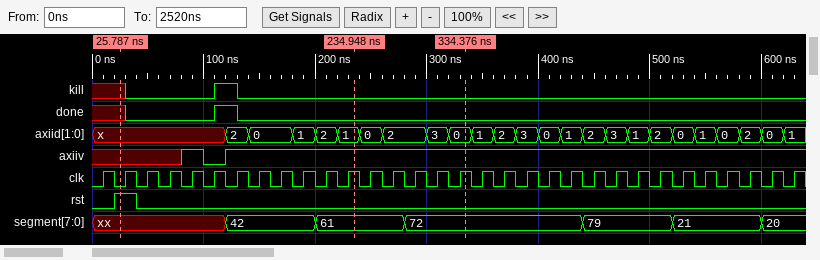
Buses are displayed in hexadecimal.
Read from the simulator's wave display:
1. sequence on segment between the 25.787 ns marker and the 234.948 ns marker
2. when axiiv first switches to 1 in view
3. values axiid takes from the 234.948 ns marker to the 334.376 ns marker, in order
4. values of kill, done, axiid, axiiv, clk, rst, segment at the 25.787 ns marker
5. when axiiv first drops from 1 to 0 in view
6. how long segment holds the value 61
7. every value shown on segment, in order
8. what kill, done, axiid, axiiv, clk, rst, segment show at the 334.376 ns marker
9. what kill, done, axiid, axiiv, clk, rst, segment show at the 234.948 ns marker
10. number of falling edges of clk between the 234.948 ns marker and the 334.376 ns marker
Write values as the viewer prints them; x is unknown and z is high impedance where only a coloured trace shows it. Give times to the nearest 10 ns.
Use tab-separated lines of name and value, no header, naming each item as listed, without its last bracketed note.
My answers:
sequence on segment between the 25.787 ns marker and the 234.948 ns marker	xx, 42, 61
when axiiv first switches to 1 in view	80 ns
values axiid takes from the 234.948 ns marker to the 334.376 ns marker, in order	1, 0, 2, 3, 0
values of kill, done, axiid, axiiv, clk, rst, segment at the 25.787 ns marker	kill=x, done=x, axiid=x, axiiv=x, clk=0, rst=1, segment=xx
when axiiv first drops from 1 to 0 in view	100 ns
how long segment holds the value 61	80 ns
every value shown on segment, in order	xx, 42, 61, 72, 79, 21, 20
what kill, done, axiid, axiiv, clk, rst, segment show at the 334.376 ns marker	kill=0, done=0, axiid=0, axiiv=1, clk=1, rst=0, segment=72
what kill, done, axiid, axiiv, clk, rst, segment show at the 234.948 ns marker	kill=0, done=0, axiid=1, axiiv=1, clk=1, rst=0, segment=61
number of falling edges of clk between the 234.948 ns marker and the 334.376 ns marker	5
